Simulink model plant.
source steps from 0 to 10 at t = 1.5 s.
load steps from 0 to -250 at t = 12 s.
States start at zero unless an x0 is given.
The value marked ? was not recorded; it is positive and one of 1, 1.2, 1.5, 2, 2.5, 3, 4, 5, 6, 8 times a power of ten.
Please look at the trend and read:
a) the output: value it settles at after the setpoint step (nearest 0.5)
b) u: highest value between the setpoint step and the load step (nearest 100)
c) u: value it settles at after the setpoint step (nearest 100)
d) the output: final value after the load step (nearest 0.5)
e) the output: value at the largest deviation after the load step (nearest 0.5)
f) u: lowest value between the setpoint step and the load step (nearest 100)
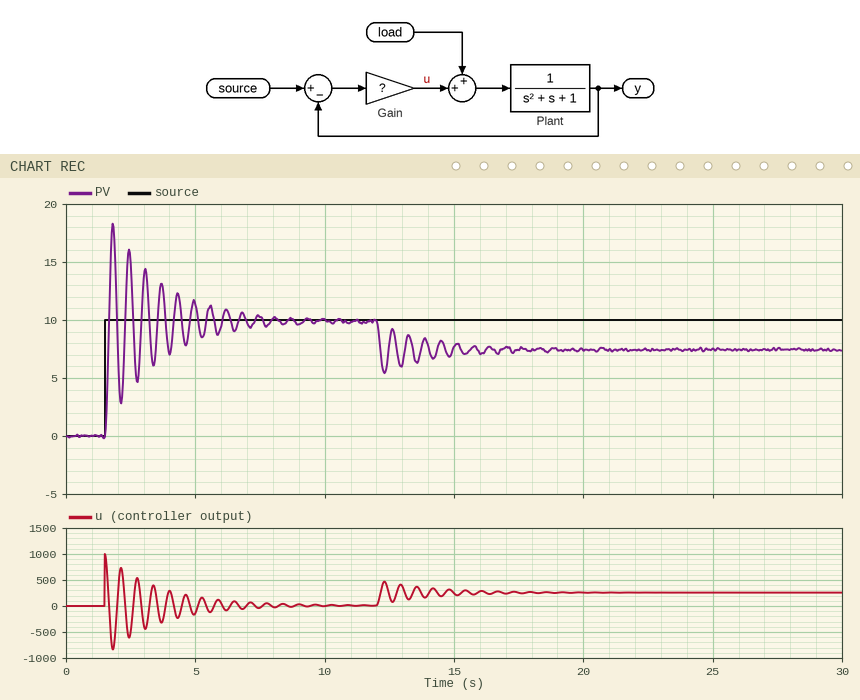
10.0
1000
0
7.5
5.5
-800
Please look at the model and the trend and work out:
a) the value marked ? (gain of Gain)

100
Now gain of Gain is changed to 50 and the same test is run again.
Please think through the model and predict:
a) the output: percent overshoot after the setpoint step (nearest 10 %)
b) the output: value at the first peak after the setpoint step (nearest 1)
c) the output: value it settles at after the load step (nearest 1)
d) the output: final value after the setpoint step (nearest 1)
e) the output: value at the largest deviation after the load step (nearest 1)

80 %
18
5
10
1
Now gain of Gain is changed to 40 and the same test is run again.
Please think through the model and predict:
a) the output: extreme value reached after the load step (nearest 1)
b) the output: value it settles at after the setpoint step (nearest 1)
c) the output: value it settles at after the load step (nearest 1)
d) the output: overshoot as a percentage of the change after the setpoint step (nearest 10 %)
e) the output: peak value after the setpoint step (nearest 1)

-1
10
4
80 %
17
